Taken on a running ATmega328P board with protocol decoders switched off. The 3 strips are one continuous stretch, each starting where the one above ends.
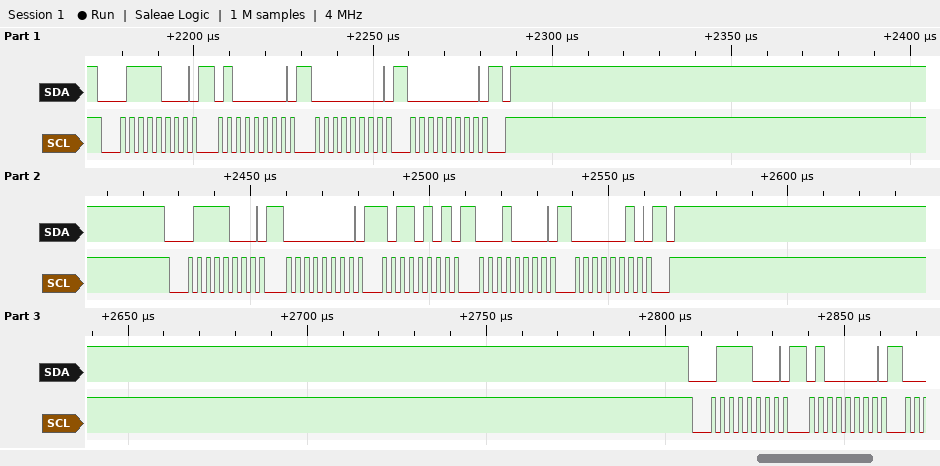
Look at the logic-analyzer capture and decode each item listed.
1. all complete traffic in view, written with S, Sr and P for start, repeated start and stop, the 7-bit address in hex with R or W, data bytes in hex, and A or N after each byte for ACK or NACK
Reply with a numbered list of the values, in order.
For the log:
1. S 3CW A 40 A 00 A 00 A P S 3CW A 00 A B5 A 10 A 02 A P S 3CW A 40 A
